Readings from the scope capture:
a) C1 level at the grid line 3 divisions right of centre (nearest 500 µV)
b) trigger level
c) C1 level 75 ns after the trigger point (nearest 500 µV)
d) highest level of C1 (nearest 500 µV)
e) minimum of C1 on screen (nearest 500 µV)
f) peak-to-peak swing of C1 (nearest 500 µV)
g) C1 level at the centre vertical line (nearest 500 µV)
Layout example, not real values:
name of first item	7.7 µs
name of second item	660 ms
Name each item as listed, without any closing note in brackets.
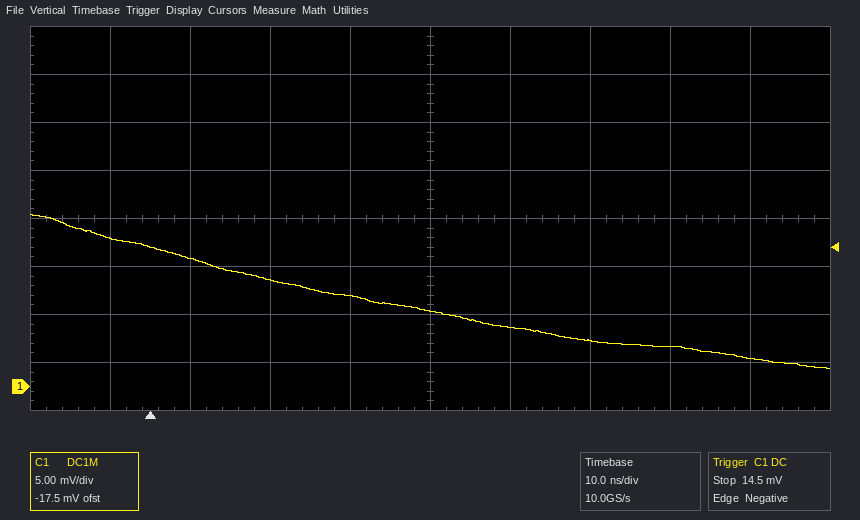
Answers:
C1 level at the grid line 3 divisions right of centre	4.0 mV
trigger level	14.5 mV
C1 level 75 ns after the trigger point	3.0 mV
highest level of C1	18.0 mV
minimum of C1 on screen	2.0 mV
peak-to-peak swing of C1	16.0 mV
C1 level at the centre vertical line	8.0 mV
